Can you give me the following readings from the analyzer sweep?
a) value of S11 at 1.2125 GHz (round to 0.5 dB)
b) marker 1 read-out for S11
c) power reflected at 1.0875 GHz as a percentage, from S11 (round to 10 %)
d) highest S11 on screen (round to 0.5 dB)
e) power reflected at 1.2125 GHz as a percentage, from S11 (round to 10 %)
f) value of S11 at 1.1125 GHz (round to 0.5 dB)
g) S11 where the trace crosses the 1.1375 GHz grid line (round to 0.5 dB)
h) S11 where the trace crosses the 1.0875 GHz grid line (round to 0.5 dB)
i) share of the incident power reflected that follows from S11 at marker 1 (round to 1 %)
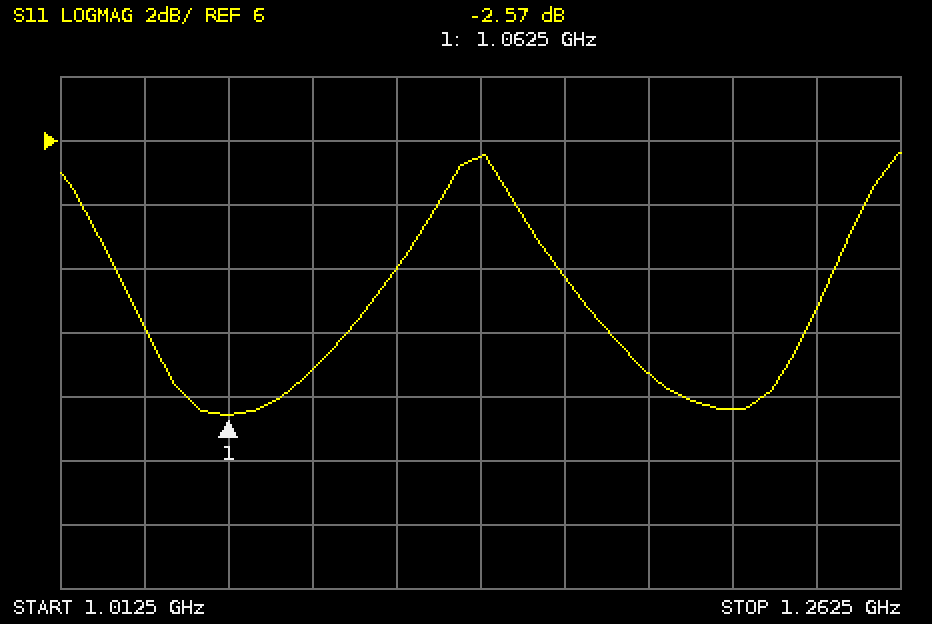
-2.5 dB
-2.57 dB
80 %
5.5 dB
60 %
2.0 dB
5.5 dB
-1.0 dB
55 %
